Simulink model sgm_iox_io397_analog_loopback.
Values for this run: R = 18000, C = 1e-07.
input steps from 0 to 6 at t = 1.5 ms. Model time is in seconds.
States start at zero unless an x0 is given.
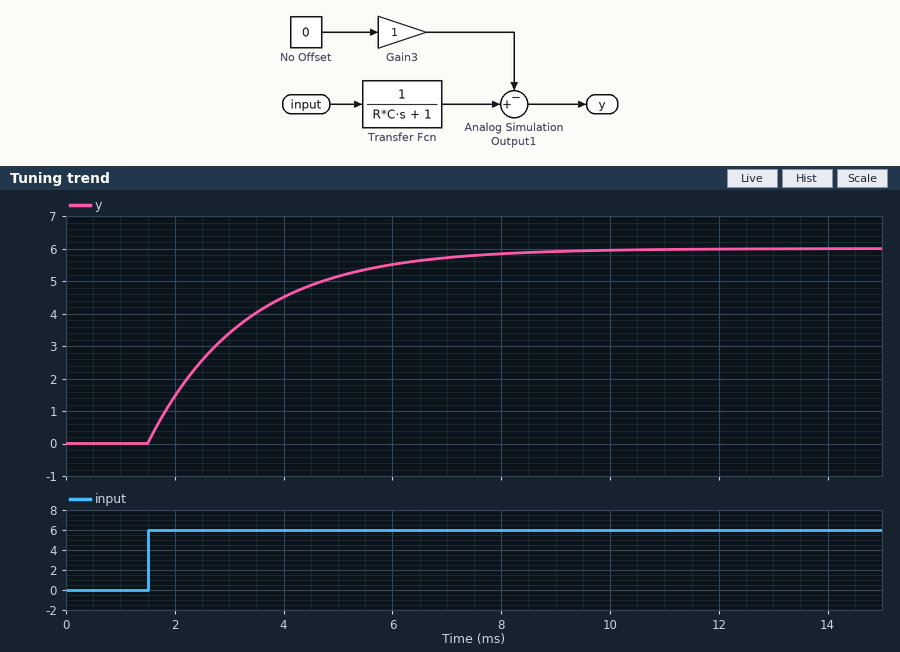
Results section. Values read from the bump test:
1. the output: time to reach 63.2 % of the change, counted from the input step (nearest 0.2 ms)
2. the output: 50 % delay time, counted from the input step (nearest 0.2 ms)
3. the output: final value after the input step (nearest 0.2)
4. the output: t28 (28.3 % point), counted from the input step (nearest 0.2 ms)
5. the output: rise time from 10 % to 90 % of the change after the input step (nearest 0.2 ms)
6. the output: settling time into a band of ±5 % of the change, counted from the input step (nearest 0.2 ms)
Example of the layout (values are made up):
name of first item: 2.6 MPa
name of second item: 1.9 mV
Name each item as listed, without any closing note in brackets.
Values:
the output: time to reach 63.2 % of the change, counted from the input step: 1.8 ms
the output: 50 % delay time, counted from the input step: 1.2 ms
the output: final value after the input step: 6.0
the output: t28 (28.3 % point), counted from the input step: 0.6 ms
the output: rise time from 10 % to 90 % of the change after the input step: 4.0 ms
the output: settling time into a band of ±5 % of the change, counted from the input step: 5.4 ms
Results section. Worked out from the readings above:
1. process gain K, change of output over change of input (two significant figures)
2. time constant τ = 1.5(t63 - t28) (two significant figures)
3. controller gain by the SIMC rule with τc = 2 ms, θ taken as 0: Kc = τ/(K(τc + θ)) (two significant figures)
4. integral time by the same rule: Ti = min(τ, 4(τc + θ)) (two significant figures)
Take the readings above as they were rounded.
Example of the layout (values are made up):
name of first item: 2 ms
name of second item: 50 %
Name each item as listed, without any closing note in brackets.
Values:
process gain K, change of output over change of input: 1.0
time constant τ = 1.5(t63 - t28): 1.8 ms
controller gain by the SIMC rule with τc = 2 ms, θ taken as 0: Kc = τ/(K(τc + θ)): 0.90
integral time by the same rule: Ti = min(τ, 4(τc + θ)): 1.8 ms
